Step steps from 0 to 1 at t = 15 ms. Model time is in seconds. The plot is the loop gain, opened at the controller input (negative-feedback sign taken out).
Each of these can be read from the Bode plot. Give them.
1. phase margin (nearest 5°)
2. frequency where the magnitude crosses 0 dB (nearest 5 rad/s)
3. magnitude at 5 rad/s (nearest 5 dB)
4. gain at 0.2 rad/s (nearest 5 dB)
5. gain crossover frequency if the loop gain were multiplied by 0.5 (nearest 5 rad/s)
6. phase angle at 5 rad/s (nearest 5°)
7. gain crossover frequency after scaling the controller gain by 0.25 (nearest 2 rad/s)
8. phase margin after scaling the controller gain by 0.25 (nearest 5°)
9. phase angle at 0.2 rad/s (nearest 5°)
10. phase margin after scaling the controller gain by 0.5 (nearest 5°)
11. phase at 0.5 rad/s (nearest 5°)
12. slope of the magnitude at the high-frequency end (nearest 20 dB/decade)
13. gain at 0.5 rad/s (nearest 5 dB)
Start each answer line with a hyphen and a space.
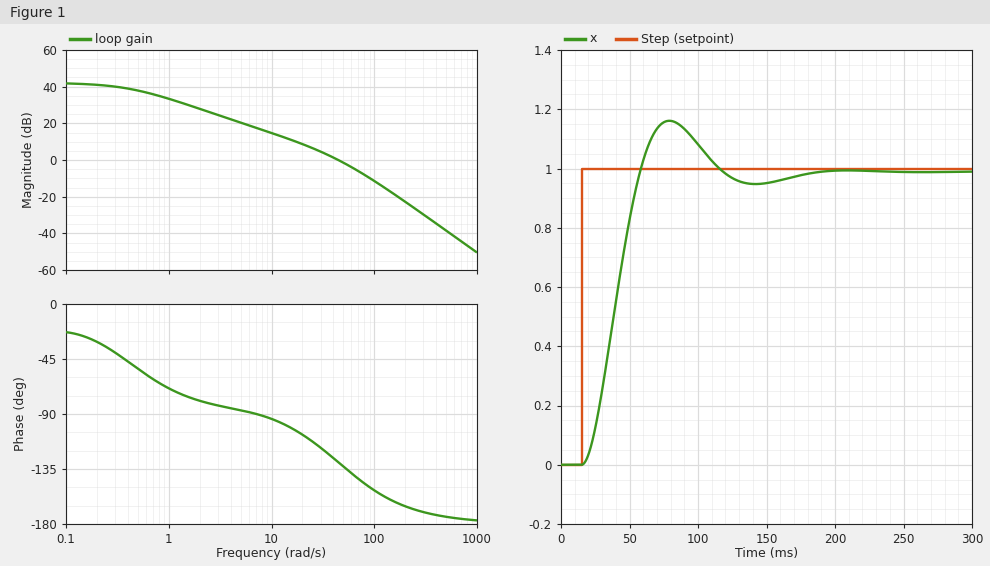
- 50°
- 45 rad/s
- 20 dB
- 40 dB
- 25 rad/s
- -85°
- 14 rad/s
- 80°
- -30°
- 65°
- -55°
- -40 dB/decade
- 40 dB
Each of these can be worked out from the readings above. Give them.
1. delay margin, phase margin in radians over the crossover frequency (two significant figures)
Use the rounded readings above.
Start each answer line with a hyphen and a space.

- 0.019 s
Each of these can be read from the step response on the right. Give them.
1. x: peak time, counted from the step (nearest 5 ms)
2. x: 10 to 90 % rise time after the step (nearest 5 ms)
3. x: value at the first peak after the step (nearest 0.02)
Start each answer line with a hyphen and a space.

- 65 ms
- 30 ms
- 1.16
